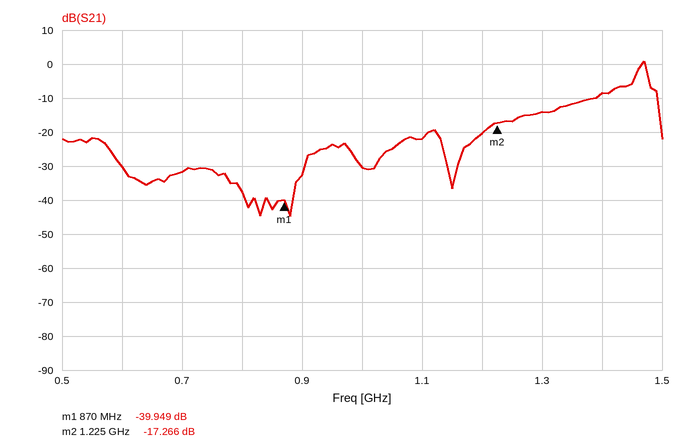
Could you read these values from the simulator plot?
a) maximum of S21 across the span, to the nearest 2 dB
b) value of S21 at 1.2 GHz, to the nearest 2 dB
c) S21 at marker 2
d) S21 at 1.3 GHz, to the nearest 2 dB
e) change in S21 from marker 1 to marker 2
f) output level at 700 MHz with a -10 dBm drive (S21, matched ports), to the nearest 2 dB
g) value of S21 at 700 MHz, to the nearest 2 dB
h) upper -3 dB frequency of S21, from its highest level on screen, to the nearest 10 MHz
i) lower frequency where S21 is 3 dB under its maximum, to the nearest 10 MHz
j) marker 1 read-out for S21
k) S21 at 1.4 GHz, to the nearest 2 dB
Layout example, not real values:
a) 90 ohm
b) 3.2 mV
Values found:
a) 0 dB
b) -20 dB
c) -17.266 dB
d) -14 dB
e) 22.683 dB
f) -42 dBm
g) -32 dB
h) 1.47 GHz
i) 1.46 GHz
j) -39.949 dB
k) -8 dB
